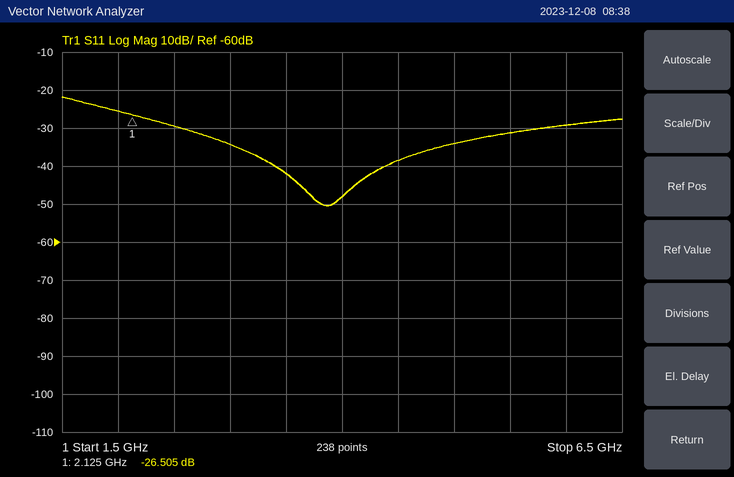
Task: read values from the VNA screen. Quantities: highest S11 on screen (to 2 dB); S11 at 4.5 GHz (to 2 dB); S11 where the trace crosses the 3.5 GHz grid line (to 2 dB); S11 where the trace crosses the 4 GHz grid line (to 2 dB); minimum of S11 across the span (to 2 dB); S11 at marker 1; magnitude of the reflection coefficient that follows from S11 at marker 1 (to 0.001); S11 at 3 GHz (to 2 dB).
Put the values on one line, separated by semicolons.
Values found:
-22 dB; -38 dB; -42 dB; -48 dB; -50 dB; -26.505 dB; 0.047; -34 dB
